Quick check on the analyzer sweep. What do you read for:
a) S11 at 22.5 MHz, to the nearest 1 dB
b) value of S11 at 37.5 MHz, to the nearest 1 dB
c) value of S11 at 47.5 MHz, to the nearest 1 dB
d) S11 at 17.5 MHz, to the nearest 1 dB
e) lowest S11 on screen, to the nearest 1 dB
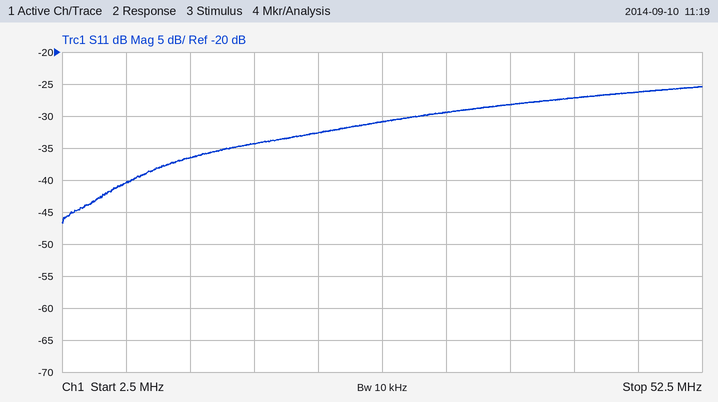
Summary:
-33 dB
-28 dB
-26 dB
-34 dB
-47 dB
